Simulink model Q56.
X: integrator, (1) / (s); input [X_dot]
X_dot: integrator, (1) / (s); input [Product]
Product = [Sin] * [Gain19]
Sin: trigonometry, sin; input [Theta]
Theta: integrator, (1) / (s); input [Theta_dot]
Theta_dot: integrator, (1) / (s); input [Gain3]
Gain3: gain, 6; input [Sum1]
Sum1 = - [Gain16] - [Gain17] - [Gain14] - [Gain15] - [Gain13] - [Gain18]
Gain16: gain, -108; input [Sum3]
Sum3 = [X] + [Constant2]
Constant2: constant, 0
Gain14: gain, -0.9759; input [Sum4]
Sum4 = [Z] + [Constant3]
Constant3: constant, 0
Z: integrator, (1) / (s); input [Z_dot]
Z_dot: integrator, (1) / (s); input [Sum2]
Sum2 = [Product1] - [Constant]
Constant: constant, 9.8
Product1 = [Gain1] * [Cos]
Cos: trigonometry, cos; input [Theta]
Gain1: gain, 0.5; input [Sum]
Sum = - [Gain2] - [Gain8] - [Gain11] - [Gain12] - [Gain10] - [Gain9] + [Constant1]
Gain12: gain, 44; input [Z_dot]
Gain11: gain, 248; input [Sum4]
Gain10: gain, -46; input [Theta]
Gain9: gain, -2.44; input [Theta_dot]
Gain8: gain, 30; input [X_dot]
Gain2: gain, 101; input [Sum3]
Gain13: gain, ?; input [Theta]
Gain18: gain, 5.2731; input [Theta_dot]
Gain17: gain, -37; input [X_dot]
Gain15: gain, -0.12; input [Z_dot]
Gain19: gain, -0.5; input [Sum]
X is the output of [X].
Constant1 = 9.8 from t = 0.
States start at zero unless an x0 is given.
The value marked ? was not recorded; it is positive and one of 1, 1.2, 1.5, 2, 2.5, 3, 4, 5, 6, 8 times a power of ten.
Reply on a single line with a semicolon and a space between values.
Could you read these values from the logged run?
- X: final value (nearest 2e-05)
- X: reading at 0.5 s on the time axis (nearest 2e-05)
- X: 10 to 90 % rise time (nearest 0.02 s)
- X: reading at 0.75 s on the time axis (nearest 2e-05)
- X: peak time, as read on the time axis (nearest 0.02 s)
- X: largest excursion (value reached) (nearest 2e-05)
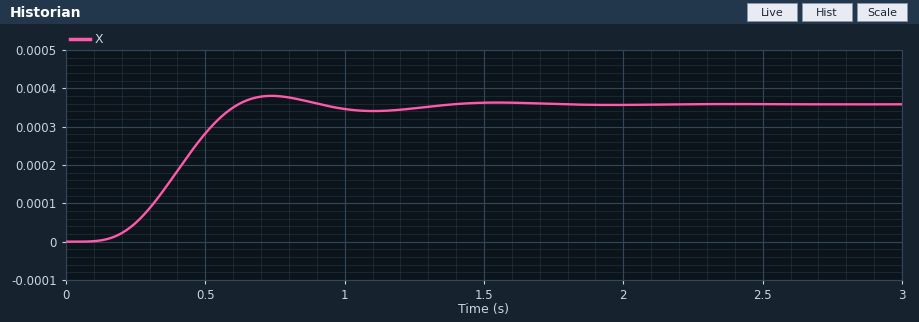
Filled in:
0.00036; 0.00028; 0.32 s; 0.00038; 0.74 s; 0.00038
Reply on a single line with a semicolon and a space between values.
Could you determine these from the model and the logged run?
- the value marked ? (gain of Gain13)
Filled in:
50
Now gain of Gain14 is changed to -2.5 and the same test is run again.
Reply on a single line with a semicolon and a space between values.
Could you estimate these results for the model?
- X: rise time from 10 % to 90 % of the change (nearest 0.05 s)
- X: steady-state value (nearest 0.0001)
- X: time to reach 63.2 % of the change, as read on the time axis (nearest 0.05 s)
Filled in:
0.40 s; 0.0009; 0.50 s
